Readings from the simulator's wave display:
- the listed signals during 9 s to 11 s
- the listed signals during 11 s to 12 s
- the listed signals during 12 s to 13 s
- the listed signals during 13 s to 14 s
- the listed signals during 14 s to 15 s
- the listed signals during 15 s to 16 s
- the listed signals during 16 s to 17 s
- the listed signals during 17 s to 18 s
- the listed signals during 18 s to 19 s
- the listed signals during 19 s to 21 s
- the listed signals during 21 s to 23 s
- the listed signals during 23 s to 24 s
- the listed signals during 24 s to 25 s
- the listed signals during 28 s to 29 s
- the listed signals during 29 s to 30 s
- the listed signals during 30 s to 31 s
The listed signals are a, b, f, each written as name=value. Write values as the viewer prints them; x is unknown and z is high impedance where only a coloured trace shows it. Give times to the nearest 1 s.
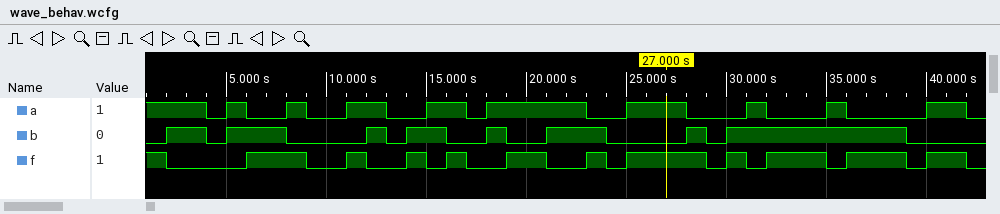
a=0, b=0, f=0
a=1, b=0, f=1
a=1, b=1, f=0
a=0, b=0, f=0
a=0, b=1, f=1
a=1, b=1, f=0
a=1, b=0, f=1
a=0, b=0, f=0
a=1, b=1, f=0
a=1, b=0, f=1
a=1, b=1, f=0
a=0, b=1, f=1
a=0, b=0, f=0
a=0, b=1, f=1
a=0, b=0, f=0
a=0, b=1, f=1
